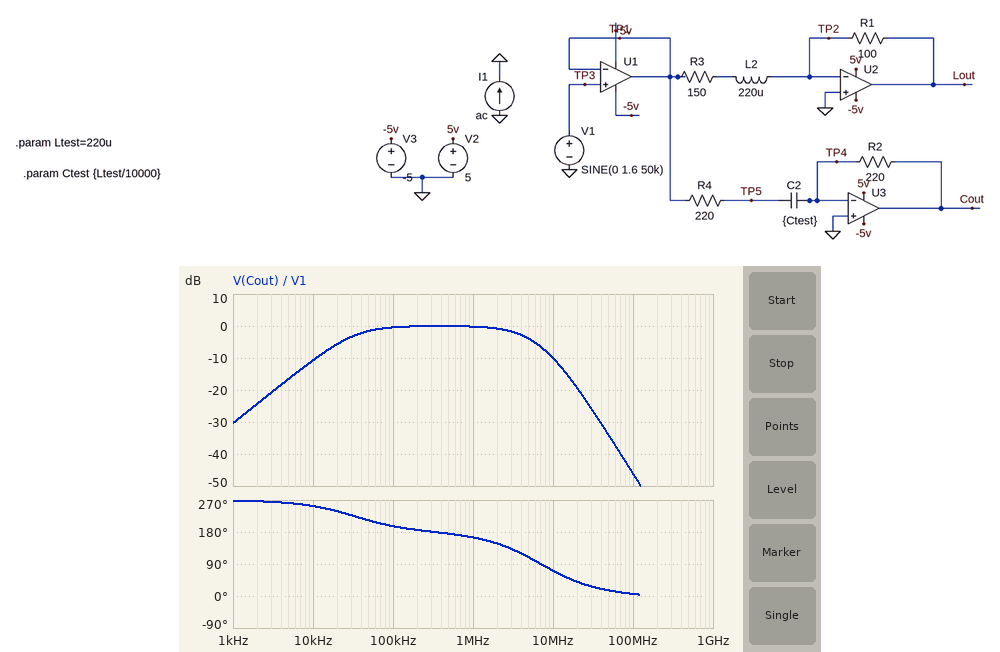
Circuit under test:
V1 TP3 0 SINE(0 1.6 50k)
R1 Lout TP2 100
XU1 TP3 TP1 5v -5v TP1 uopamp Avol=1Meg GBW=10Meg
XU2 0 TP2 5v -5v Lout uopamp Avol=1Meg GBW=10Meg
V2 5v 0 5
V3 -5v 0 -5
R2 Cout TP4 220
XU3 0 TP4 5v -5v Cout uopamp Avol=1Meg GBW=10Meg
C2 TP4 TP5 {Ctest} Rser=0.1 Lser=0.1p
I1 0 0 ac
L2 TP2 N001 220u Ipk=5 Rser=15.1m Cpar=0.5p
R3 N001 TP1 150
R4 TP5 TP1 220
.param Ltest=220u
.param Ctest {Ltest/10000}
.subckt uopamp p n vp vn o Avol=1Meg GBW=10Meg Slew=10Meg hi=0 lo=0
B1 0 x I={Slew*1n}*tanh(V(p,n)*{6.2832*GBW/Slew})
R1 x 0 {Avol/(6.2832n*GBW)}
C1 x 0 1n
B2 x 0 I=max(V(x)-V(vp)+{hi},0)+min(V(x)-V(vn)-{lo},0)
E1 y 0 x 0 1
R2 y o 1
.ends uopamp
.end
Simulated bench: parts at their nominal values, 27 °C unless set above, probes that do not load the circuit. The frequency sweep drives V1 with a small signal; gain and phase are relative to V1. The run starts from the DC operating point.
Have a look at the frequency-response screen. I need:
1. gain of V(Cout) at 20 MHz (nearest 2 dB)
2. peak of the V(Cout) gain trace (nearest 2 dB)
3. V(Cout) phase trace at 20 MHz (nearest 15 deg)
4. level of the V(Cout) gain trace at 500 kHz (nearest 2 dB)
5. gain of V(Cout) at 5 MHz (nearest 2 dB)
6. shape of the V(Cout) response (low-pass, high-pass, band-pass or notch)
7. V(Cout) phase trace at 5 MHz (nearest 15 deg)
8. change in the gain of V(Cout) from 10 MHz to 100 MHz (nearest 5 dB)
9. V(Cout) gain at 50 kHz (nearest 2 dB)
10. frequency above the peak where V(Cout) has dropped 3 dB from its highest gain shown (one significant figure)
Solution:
-20 dB
0 dB
45 deg
0 dB
-4 dB
band-pass
105 deg
-35 dB
-2 dB
4 MHz
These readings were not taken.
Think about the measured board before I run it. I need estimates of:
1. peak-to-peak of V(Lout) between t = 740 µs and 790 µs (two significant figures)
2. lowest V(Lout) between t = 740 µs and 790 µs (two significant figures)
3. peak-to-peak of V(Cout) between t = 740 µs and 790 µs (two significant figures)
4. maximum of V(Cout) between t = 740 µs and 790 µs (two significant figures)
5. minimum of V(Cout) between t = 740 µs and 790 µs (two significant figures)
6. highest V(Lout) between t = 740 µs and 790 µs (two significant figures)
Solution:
1.9 V
-970 mV
2.7 V
1.3 V
-1.3 V
970 mV
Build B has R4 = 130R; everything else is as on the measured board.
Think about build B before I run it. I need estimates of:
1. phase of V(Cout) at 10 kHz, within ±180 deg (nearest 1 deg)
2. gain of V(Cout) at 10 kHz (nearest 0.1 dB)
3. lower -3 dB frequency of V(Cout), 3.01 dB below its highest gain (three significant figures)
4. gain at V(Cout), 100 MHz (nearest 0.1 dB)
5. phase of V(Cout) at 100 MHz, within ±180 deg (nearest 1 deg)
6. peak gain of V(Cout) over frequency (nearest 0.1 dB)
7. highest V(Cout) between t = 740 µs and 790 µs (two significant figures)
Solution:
-100 deg
-10.5 dB
54.4 kHz
-44.1 dB
5 deg
4.5 dB
1.8 V
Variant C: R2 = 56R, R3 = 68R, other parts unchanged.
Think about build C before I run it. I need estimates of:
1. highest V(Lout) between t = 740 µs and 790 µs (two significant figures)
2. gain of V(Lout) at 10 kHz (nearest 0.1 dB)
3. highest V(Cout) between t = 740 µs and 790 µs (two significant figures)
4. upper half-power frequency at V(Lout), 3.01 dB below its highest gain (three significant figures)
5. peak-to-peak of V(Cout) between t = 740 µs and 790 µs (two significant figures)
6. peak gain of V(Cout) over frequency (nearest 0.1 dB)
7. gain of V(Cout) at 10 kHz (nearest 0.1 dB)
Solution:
1.6 V
3.2 dB
340 mV
48.8 kHz
680 mV
-11.9 dB
-22.6 dB
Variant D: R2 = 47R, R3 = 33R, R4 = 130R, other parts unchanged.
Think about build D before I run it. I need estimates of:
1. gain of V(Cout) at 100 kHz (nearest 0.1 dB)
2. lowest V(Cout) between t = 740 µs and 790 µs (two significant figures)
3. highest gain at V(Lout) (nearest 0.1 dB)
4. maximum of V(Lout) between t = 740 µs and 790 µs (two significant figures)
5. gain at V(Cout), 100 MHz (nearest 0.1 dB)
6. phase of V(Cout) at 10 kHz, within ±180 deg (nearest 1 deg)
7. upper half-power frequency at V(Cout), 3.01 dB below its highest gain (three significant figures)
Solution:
-10.0 dB
-390 mV
9.6 dB
2.1 V
-51.5 dB
-100 deg
5.47 MHz
